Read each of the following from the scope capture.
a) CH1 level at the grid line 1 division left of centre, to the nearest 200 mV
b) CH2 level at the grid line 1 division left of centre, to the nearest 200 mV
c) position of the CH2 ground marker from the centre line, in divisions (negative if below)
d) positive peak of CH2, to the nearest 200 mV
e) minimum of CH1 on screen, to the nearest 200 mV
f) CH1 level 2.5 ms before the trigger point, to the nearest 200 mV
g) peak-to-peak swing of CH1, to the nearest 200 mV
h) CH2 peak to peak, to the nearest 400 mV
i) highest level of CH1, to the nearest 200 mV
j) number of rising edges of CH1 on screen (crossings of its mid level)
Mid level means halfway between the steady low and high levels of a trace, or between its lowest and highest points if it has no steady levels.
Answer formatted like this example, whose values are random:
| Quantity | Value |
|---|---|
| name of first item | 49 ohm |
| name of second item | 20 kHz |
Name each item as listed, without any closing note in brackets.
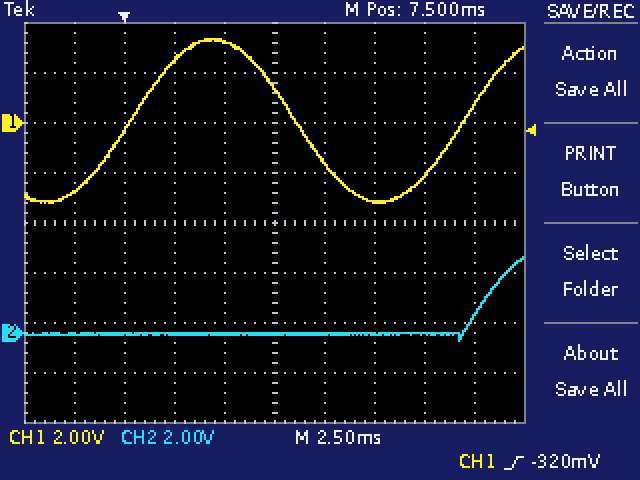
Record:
| Quantity | Value |
|---|---|
| CH1 level at the grid line 1 division left of centre, to the nearest 200 mV | 3.2 V |
| CH2 level at the grid line 1 division left of centre, to the nearest 200 mV | 0.0 V |
| position of the CH2 ground marker from the centre line, in divisions | -2.2 div |
| positive peak of CH2, to the nearest 200 mV | 3.0 V |
| minimum of CH1 on screen, to the nearest 200 mV | -3.2 V |
| CH1 level 2.5 ms before the trigger point, to the nearest 200 mV | -2.8 V |
| peak-to-peak swing of CH1, to the nearest 200 mV | 6.6 V |
| CH2 peak to peak, to the nearest 400 mV | 3.2 V |
| highest level of CH1, to the nearest 200 mV | 3.4 V |
| number of rising edges of CH1 on screen | 2 |
